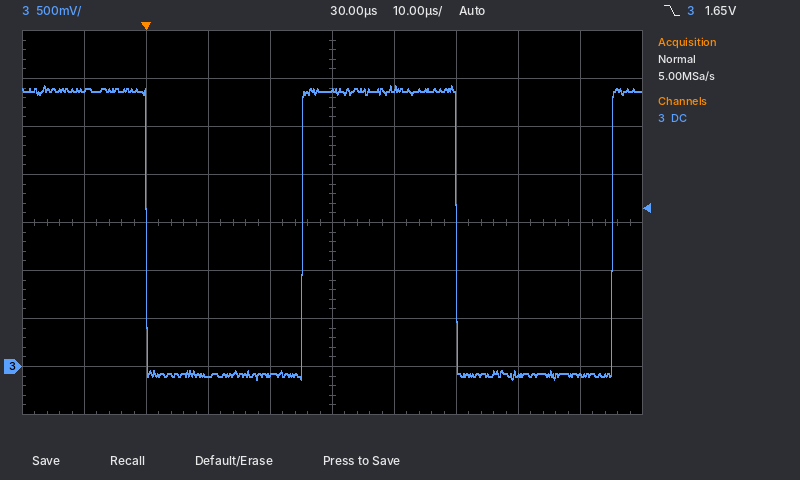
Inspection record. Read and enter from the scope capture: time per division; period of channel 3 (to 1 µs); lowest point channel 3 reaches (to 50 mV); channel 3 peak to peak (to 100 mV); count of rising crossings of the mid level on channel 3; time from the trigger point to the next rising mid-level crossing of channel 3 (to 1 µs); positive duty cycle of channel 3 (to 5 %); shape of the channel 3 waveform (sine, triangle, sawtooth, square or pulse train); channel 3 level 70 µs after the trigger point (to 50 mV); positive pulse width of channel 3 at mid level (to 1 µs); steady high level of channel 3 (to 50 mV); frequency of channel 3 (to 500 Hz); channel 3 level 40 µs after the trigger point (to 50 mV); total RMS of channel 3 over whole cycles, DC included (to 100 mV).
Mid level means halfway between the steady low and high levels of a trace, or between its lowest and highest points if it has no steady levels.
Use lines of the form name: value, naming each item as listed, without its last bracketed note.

time per division: 10 µs
period of channel 3: 50 µs
lowest point channel 3 reaches: -150 mV
channel 3 peak to peak: 3.10 V
count of rising crossings of the mid level on channel 3: 2
time from the trigger point to the next rising mid-level crossing of channel 3: 25 µs
positive duty cycle of channel 3: 50 %
shape of the channel 3 waveform: square
channel 3 level 70 µs after the trigger point: -100 mV
positive pulse width of channel 3 at mid level: 25 µs
steady high level of channel 3: 2.85 V
frequency of channel 3: 20.0 kHz
channel 3 level 40 µs after the trigger point: 2.90 V
total RMS of channel 3 over whole cycles, DC included: 2.0 V
